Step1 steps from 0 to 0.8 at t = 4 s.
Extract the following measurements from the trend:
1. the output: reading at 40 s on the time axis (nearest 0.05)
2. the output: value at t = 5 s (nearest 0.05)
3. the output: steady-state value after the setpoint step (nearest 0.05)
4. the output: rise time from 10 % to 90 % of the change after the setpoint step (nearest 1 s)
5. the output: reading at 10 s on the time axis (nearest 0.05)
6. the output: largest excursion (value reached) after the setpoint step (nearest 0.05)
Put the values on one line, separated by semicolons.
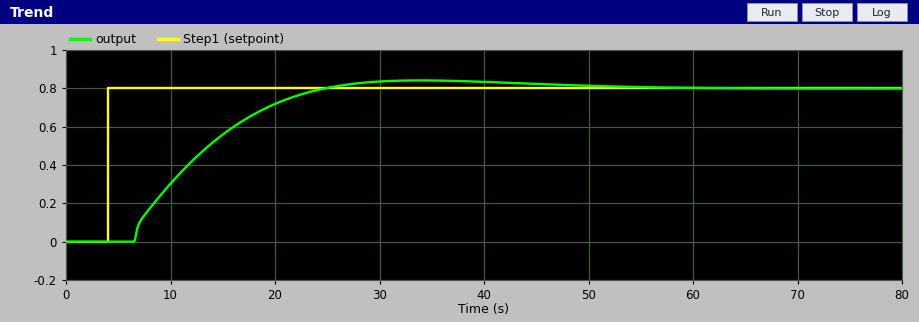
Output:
0.85; 0.00; 0.80; 13 s; 0.30; 0.85
